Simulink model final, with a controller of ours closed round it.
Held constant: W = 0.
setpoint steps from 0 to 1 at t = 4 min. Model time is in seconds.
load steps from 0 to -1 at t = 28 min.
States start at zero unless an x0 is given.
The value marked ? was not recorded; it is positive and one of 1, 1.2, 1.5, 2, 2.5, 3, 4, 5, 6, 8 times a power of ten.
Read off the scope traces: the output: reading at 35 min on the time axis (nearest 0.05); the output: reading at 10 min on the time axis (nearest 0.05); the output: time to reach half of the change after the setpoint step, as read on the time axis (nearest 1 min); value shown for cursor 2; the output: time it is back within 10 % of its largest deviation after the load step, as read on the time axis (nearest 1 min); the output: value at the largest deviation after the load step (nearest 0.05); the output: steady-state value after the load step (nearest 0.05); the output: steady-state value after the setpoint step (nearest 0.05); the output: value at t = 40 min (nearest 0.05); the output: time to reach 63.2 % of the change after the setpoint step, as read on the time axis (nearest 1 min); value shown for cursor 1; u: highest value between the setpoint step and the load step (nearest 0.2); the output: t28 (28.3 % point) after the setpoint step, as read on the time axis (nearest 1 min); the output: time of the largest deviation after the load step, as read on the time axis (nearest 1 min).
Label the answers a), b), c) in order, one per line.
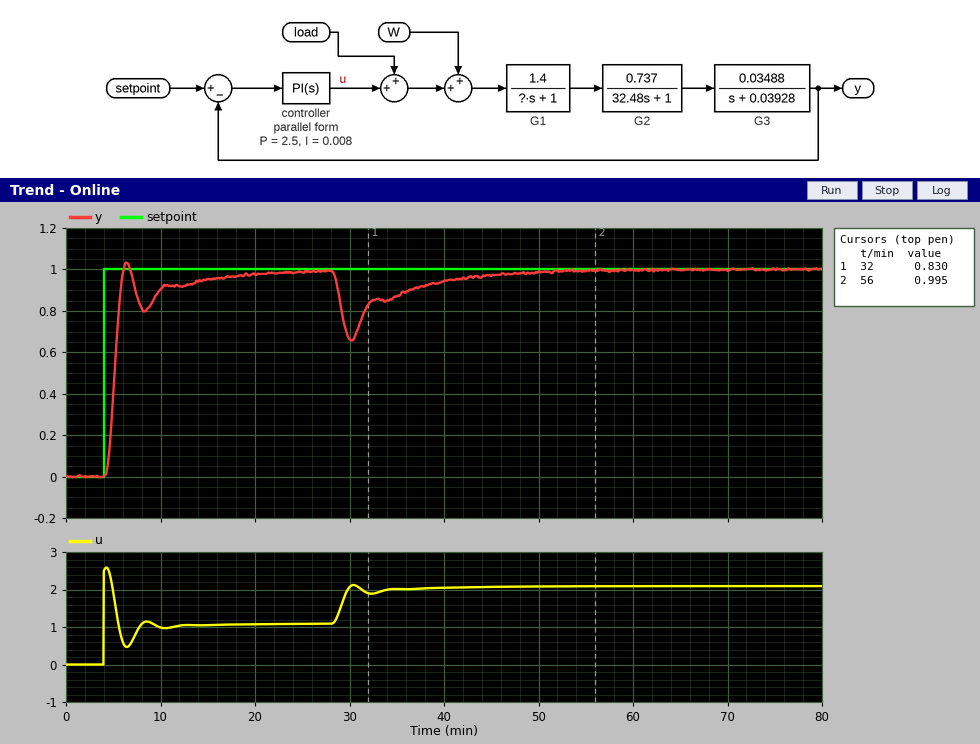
a) 0.85
b) 0.90
c) 5 min
d) 0.995
e) 44 min
f) 0.65
g) 1.00
h) 1.00
i) 0.95
j) 5 min
k) 0.830
l) 2.6
m) 5 min
n) 30 min
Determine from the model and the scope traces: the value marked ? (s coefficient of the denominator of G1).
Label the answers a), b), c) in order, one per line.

a) 80
